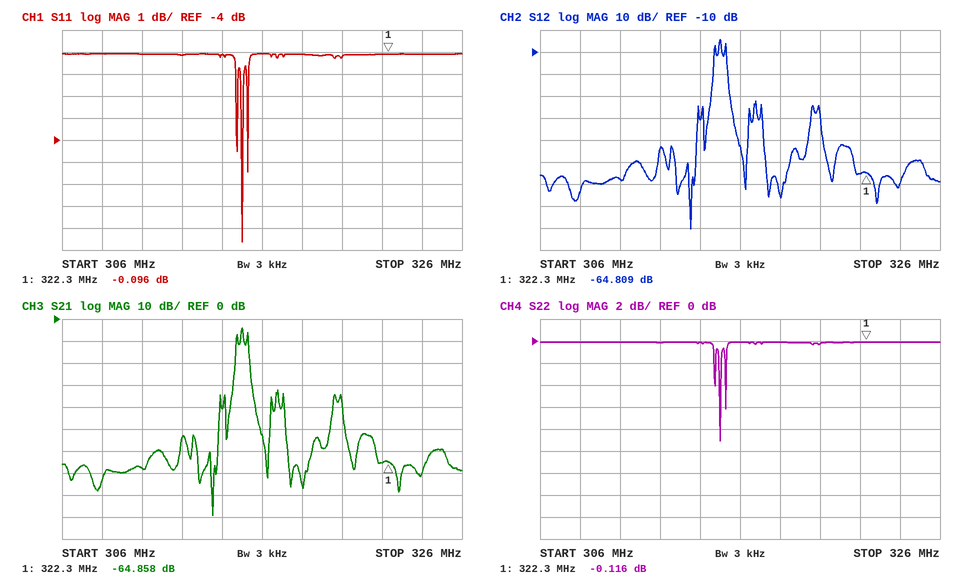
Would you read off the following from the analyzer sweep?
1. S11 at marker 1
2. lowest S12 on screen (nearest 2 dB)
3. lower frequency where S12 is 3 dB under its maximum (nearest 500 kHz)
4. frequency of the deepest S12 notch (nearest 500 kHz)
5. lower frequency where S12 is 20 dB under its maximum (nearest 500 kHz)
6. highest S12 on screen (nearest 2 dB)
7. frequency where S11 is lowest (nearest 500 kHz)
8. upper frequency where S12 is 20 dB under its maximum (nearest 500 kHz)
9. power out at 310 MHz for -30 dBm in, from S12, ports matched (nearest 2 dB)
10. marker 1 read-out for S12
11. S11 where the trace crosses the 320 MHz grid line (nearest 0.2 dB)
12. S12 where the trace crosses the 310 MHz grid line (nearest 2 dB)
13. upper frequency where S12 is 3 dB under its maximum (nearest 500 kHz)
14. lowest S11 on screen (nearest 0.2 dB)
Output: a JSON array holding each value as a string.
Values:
["-0.096 dB", "-90 dB", "315.0 MHz", "313.5 MHz", "314.5 MHz", "-4 dB", "315.0 MHz", "315.5 MHz", "-98 dBm", "-64.809 dB", "-0.2 dB", "-68 dB", "315.0 MHz", "-8.6 dB"]
